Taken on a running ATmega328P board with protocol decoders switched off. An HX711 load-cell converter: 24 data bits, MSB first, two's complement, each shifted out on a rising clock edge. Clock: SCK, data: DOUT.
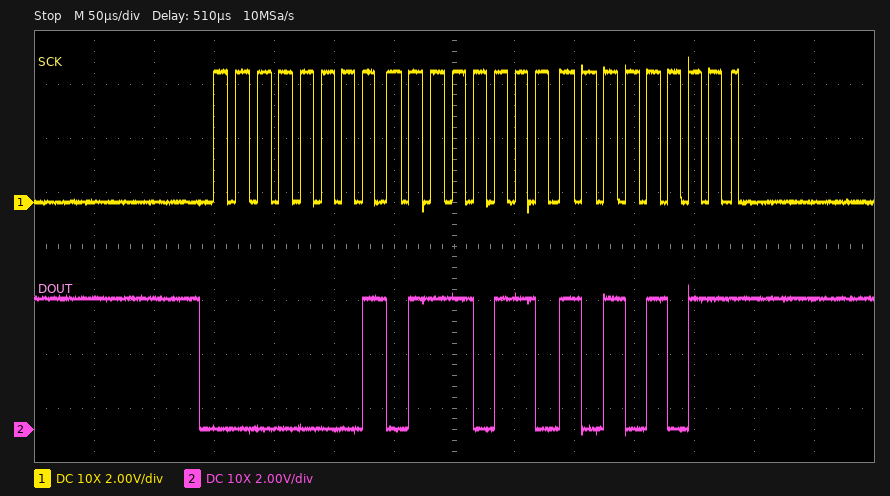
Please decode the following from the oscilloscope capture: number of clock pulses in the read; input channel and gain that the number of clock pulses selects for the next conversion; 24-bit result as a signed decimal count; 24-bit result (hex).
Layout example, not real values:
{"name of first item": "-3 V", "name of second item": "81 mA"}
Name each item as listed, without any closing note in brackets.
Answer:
{"number of clock pulses in the read": "25", "input channel and gain that the number of clock pulses selects for the next conversion": "channel A, gain 128", "24-bit result as a signed decimal count": "95915", "24-bit result": "0x0176AB"}
